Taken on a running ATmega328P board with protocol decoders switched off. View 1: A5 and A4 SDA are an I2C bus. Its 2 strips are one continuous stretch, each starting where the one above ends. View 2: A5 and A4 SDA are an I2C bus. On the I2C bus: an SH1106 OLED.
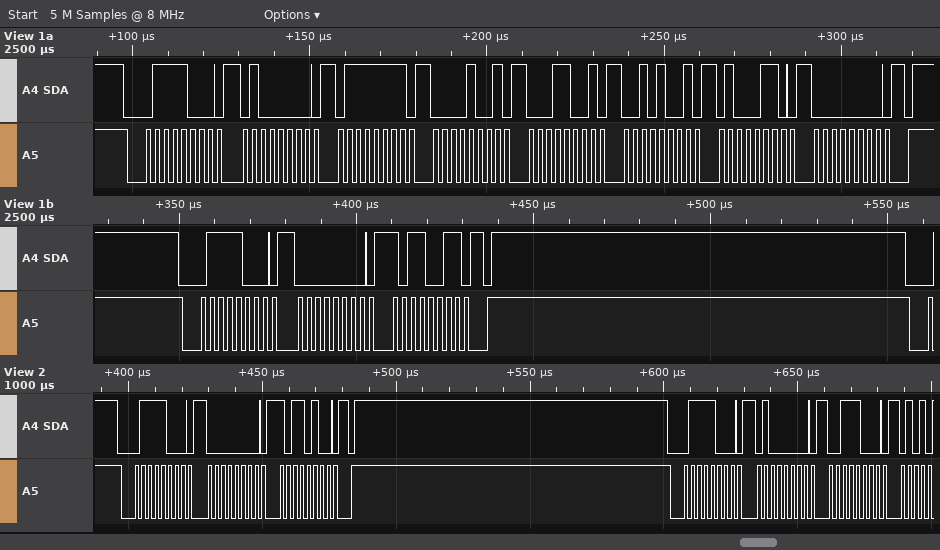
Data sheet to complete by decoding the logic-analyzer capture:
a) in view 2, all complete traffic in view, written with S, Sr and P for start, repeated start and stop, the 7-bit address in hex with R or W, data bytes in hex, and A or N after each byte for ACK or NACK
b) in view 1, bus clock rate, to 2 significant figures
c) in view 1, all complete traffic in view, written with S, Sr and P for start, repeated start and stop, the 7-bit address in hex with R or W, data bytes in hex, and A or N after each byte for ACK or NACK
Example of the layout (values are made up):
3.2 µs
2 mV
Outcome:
S 3CW A 00 A B4 A P S 3CW A 40 A 38 A
400 kHz
S 3CW A 40 A 7F A 09 A 19 A 29 A 46 A 00 A P S 3CW A 00 A B3 A P
